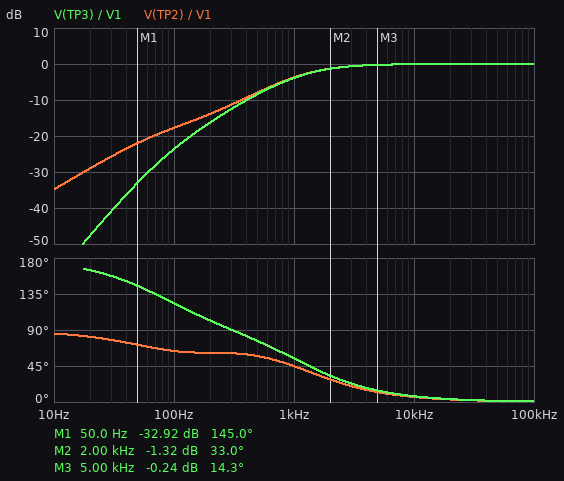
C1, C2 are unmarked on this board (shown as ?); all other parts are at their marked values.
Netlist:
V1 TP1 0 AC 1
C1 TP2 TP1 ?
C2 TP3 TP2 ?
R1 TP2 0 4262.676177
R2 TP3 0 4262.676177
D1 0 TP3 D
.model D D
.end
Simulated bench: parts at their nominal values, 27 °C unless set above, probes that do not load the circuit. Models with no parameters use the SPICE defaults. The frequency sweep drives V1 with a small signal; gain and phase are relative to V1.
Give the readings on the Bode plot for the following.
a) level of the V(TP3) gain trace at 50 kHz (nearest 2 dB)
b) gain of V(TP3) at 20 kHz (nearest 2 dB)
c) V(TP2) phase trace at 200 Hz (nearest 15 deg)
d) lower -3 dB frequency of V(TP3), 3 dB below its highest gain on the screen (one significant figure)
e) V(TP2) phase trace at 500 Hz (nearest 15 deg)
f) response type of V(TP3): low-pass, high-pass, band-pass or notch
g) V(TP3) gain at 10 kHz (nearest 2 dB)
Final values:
0 dB
0 dB
60 deg
1 kHz
60 deg
high-pass
0 dB
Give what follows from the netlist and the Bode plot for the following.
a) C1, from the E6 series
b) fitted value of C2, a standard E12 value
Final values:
68 nF
220 nF
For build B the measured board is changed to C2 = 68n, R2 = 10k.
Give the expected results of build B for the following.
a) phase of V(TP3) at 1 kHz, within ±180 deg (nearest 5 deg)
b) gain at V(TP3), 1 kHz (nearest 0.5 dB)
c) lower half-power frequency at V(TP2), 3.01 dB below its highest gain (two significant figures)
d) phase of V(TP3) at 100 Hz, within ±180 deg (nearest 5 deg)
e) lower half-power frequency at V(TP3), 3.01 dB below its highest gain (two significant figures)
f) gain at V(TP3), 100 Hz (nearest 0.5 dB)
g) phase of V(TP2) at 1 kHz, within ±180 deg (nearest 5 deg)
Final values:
50 deg
-2.5 dB
830 Hz
140 deg
890 Hz
-24.0 dB
35 deg
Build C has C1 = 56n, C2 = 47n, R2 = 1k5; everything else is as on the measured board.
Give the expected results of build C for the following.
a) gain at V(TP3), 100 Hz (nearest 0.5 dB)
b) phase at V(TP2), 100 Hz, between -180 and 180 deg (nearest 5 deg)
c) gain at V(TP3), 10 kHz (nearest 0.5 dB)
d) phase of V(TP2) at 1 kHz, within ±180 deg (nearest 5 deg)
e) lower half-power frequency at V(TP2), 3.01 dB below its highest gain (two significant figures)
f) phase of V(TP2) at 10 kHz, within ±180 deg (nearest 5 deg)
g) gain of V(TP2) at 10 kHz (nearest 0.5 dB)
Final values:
-44.0 dB
75 deg
-1.0 dB
30 deg
3.2 kHz
15 deg
-0.5 dB
